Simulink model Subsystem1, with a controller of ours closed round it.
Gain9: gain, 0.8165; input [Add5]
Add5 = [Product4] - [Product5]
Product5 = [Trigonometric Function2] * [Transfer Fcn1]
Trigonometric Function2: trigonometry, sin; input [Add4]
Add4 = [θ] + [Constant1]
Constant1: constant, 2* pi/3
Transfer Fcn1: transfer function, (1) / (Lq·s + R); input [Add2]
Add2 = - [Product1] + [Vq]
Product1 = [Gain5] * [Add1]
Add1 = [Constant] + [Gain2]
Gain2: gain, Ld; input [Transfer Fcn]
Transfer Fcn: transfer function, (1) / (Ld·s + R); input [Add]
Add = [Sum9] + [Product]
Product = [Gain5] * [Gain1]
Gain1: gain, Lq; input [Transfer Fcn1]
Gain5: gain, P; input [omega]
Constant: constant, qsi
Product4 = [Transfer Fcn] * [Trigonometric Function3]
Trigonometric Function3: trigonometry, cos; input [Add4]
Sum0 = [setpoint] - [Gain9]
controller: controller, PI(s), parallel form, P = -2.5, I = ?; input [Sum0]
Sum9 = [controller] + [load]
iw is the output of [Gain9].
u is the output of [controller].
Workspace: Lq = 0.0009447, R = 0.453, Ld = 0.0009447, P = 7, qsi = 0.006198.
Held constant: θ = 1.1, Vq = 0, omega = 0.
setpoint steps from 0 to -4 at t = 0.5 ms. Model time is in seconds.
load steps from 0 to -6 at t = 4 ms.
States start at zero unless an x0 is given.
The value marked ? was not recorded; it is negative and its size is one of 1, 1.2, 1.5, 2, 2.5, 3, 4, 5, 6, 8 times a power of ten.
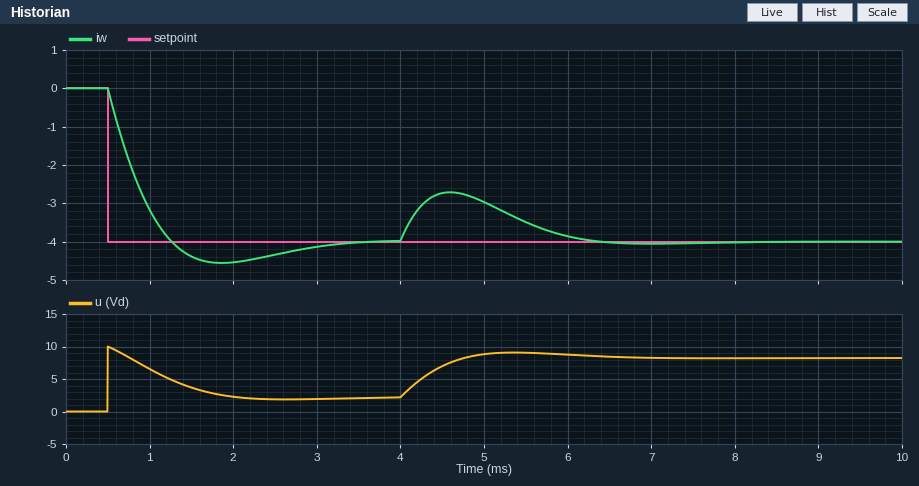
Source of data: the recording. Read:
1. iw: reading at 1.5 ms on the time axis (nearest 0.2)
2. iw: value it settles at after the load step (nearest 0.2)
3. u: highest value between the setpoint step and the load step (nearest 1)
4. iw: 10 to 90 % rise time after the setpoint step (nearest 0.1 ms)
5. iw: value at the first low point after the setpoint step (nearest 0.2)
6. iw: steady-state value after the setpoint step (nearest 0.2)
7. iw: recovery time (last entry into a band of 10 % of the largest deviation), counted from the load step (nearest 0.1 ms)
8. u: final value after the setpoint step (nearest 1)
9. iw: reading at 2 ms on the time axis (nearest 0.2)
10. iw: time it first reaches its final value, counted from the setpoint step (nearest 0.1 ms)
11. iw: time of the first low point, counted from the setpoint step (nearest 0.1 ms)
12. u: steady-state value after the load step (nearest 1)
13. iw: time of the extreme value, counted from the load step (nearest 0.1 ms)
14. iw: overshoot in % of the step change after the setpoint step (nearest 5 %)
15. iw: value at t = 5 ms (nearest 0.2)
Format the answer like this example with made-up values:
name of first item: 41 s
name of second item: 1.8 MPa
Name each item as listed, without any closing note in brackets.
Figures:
iw: reading at 1.5 ms on the time axis: -4.4
iw: value it settles at after the load step: -4.0
u: highest value between the setpoint step and the load step: 10
iw: 10 to 90 % rise time after the setpoint step: 0.6 ms
iw: value at the first low point after the setpoint step: -4.6
iw: steady-state value after the setpoint step: -4.0
iw: recovery time (last entry into a band of 10 % of the largest deviation), counted from the load step: 2.0 ms
u: final value after the setpoint step: 2
iw: reading at 2 ms on the time axis: -4.6
iw: time it first reaches its final value, counted from the setpoint step: 0.8 ms
iw: time of the first low point, counted from the setpoint step: 1.4 ms
u: steady-state value after the load step: 8
iw: time of the extreme value, counted from the load step: 0.6 ms
iw: overshoot in % of the step change after the setpoint step: 15 %
iw: value at t = 5 ms: -3.0
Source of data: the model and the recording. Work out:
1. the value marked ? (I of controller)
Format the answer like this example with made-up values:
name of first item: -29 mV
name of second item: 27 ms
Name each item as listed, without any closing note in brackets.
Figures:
the value marked ?: -4000
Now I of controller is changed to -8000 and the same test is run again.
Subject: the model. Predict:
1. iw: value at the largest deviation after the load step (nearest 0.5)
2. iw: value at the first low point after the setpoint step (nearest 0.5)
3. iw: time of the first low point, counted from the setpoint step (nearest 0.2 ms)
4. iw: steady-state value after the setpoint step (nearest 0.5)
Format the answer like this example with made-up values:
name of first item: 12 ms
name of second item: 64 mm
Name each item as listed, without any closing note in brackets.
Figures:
iw: value at the largest deviation after the load step: -3.0
iw: value at the first low point after the setpoint step: -5.0
iw: time of the first low point, counted from the setpoint step: 1.0 ms
iw: steady-state value after the setpoint step: -4.0
